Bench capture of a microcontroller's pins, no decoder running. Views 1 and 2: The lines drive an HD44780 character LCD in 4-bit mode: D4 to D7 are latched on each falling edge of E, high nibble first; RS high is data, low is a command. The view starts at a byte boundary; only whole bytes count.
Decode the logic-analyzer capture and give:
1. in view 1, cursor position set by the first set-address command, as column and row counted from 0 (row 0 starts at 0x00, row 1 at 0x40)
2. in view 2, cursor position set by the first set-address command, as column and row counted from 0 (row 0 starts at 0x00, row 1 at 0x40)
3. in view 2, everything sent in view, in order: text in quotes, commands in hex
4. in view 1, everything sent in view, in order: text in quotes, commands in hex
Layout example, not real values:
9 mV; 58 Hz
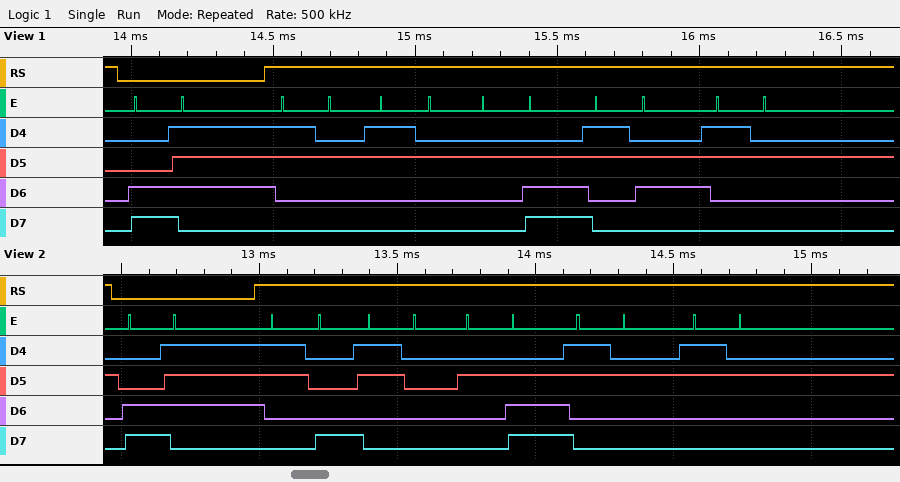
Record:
column 7, row 1; column 7, row 1; 0xC7 "80.22"; 0xC7 "22.62"
